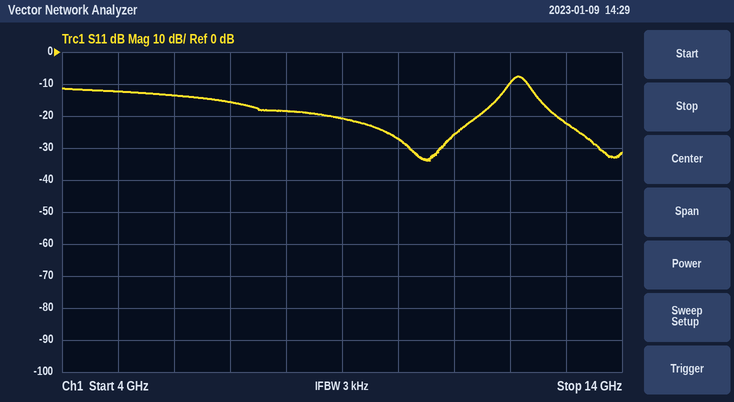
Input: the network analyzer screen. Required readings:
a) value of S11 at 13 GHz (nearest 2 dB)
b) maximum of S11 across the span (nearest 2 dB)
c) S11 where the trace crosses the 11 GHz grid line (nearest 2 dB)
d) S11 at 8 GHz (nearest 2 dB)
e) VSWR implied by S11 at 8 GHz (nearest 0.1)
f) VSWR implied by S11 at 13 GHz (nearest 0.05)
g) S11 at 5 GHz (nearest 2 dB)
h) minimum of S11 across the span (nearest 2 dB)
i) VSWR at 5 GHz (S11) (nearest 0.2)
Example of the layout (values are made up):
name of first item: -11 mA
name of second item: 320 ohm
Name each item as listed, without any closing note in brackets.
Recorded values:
value of S11 at 13 GHz: -22 dB
maximum of S11 across the span: -8 dB
S11 where the trace crosses the 11 GHz grid line: -26 dB
S11 at 8 GHz: -18 dB
VSWR implied by S11 at 8 GHz: 1.3
VSWR implied by S11 at 13 GHz: 1.15
S11 at 5 GHz: -12 dB
minimum of S11 across the span: -34 dB
VSWR at 5 GHz (S11): 1.6
